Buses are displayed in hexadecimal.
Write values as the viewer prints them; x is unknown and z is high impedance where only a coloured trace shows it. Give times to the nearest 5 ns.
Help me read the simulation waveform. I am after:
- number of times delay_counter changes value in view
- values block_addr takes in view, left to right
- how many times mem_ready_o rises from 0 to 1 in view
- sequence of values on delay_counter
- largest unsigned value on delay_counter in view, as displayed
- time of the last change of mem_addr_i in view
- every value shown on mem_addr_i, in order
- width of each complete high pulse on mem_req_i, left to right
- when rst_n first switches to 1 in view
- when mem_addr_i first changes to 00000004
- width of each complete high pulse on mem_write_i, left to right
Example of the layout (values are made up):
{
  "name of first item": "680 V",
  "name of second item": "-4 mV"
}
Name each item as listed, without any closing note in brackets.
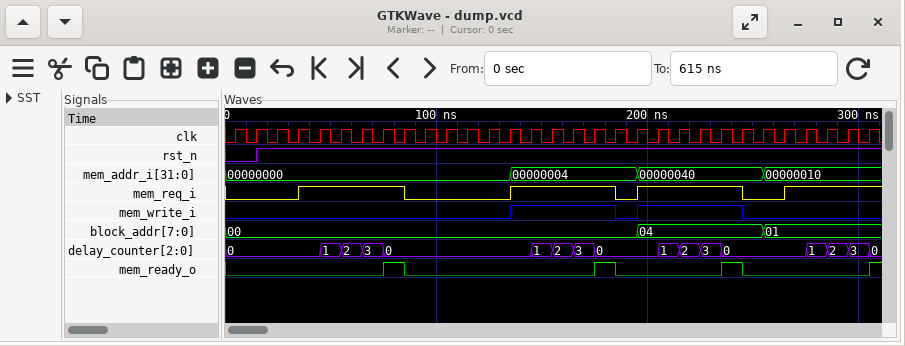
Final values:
{
  "number of times delay_counter changes value in view": "16",
  "values block_addr takes in view, left to right": "00, 04, 01",
  "how many times mem_ready_o rises from 0 to 1 in view": "4",
  "sequence of values on delay_counter": "0, 1, 2, 3, 0, 1, 2, 3, 0, 1, 2, 3, 0, 1, 2, 3, 0",
  "largest unsigned value on delay_counter in view, as displayed": "3",
  "time of the last change of mem_addr_i in view": "255 ns",
  "every value shown on mem_addr_i, in order": "00000000, 00000004, 00000040, 00000010",
  "width of each complete high pulse on mem_req_i, left to right": "50 ns, 50 ns, 50 ns",
  "when rst_n first switches to 1 in view": "15 ns",
  "when mem_addr_i first changes to 00000004": "135 ns",
  "width of each complete high pulse on mem_write_i, left to right": "50 ns, 50 ns"
}
